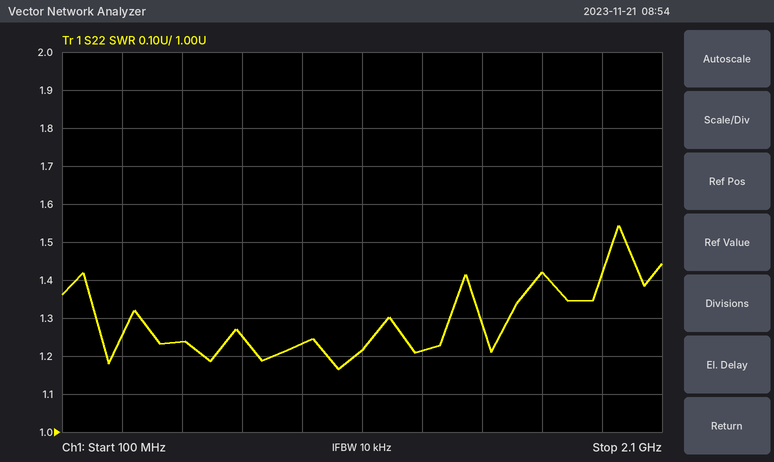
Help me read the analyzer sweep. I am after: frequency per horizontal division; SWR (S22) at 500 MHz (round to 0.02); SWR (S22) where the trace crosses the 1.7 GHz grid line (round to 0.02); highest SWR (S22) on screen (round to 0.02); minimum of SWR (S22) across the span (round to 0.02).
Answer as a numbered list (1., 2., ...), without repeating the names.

1. 200 MHz
2. 1.24
3. 1.42
4. 1.54
5. 1.16
